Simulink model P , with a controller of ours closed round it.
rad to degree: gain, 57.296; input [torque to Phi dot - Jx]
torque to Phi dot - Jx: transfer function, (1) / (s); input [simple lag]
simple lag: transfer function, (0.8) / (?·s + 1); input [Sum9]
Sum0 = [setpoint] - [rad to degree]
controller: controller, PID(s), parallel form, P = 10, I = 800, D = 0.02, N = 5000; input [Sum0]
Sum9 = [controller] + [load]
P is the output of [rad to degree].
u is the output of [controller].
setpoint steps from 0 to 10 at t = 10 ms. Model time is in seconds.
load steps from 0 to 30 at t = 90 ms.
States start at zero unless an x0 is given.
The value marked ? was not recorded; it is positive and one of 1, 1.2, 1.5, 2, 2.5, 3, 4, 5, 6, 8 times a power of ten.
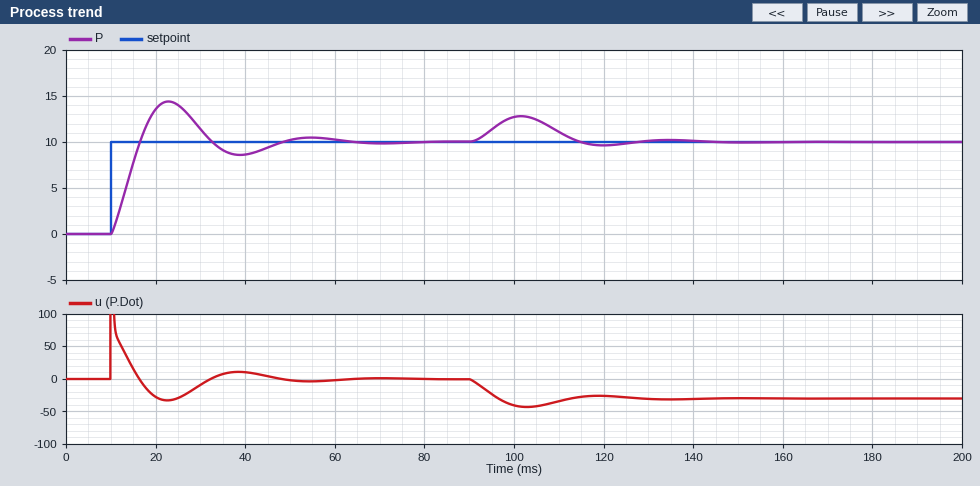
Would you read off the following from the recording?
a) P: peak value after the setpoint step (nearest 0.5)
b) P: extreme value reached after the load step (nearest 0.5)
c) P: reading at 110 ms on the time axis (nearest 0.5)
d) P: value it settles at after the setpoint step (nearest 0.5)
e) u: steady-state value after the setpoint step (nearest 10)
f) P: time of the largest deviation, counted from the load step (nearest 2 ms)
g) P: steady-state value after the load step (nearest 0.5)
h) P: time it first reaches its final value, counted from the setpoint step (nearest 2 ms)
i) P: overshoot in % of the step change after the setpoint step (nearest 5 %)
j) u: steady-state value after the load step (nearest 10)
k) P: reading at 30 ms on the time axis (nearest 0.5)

14.5
13.0
11.0
10.0
0
12 ms
10.0
6 ms
45 %
-30
11.5
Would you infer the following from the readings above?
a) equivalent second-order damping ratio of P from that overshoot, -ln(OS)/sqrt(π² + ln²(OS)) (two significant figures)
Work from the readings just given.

0.25
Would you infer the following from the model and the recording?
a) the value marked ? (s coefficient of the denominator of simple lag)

0.008
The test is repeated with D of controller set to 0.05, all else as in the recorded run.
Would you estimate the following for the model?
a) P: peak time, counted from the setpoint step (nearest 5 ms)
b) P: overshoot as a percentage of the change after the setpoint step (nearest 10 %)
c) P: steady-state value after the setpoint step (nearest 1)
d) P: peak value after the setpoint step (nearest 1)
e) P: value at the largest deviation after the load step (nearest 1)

15 ms
20 %
10
12
12
